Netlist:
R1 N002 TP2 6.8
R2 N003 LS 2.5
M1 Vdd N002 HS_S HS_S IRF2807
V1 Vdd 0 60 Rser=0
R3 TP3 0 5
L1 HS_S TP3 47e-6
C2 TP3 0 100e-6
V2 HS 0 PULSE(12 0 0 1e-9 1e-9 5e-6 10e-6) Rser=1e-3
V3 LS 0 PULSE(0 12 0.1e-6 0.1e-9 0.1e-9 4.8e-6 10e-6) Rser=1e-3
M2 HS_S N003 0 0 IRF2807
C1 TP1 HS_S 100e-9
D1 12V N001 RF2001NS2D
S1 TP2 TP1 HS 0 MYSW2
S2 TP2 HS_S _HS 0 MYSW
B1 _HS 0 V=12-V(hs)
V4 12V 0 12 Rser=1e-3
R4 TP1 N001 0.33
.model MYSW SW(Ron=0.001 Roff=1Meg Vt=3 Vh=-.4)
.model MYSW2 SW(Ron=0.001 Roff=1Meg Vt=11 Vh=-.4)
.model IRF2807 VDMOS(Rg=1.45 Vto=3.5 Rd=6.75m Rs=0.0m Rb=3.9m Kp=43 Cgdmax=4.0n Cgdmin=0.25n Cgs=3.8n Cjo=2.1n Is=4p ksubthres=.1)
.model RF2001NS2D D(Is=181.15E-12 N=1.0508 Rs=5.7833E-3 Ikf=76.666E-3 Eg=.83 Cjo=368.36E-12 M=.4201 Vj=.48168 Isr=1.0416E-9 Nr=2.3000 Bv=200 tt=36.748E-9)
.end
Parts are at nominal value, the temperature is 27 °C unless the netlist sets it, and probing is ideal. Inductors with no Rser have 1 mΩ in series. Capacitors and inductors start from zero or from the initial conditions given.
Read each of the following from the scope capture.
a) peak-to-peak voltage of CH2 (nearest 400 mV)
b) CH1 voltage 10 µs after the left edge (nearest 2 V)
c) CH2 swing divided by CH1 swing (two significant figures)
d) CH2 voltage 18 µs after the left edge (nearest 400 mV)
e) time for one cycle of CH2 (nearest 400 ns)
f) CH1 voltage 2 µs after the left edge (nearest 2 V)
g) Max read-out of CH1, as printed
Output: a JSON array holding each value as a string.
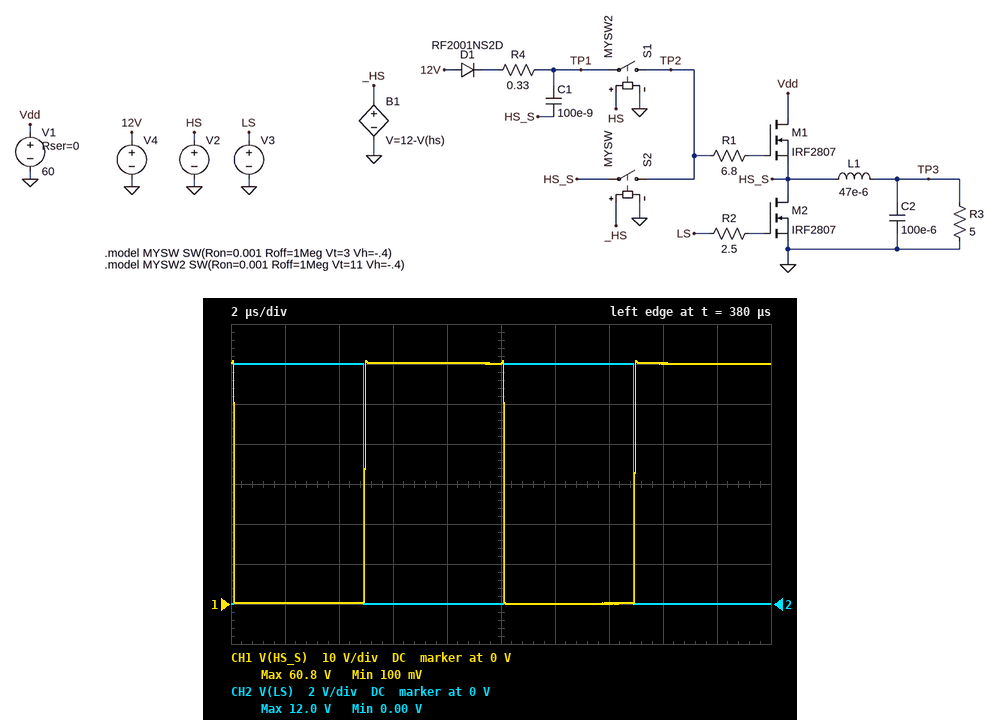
["12.0 V", "60 V", "0.20", "0 V", "10.0 µs", "0 V", "60.8 V"]
